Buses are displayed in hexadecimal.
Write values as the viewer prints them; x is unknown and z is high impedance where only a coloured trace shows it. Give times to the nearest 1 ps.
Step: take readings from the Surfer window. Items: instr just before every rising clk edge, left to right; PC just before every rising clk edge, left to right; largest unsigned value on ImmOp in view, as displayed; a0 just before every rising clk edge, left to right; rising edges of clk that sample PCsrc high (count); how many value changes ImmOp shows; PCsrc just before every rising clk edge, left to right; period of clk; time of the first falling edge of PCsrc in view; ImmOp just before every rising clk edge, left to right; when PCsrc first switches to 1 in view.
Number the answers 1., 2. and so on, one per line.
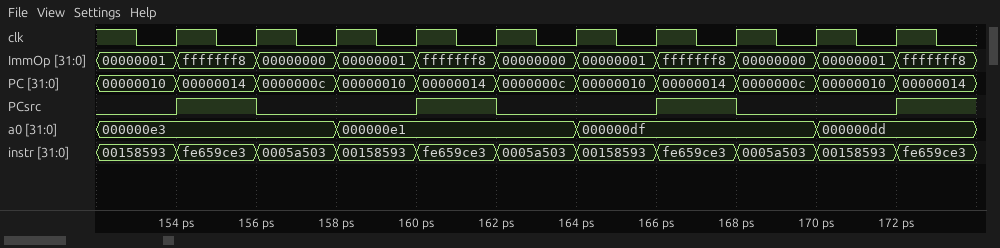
1. 00158593, fe659ce3, 0005a503, 00158593, fe659ce3, 0005a503, 00158593, fe659ce3, 0005a503, 00158593
2. 00000010, 00000014, 0000000c, 00000010, 00000014, 0000000c, 00000010, 00000014, 0000000c, 00000010
3. fffffff8
4. 000000e3, 000000e3, 000000e3, 000000e1, 000000e1, 000000e1, 000000df, 000000df, 000000df, 000000dd
5. 3
6. 10
7. 0 1 0 0 1 0 0 1 0 0
8. 2 ps
9. 156 ps
10. 00000001, fffffff8, 00000000, 00000001, fffffff8, 00000000, 00000001, fffffff8, 00000000, 00000001
11. 154 ps
